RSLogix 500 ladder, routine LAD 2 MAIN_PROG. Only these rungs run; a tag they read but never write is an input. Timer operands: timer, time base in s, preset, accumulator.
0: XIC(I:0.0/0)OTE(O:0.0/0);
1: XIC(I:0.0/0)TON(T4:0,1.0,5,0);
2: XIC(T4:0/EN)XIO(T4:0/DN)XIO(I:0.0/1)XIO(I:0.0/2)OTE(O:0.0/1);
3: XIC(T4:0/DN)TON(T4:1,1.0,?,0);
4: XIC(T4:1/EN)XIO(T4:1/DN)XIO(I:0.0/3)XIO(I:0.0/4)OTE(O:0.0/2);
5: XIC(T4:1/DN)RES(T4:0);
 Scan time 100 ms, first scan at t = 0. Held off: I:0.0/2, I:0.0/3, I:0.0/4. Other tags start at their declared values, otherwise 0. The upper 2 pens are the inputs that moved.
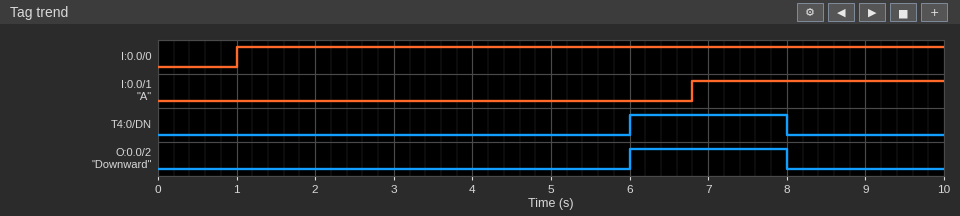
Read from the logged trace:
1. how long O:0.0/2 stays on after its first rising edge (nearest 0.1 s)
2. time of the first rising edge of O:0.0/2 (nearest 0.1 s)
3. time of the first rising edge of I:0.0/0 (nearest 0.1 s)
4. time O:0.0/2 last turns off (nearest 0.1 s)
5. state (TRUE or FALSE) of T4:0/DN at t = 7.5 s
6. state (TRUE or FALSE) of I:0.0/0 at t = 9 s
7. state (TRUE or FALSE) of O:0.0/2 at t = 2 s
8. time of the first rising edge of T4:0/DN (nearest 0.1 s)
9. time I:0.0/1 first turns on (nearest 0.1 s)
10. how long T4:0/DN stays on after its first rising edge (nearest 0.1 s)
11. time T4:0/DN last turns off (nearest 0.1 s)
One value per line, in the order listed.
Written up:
2.0 s
6.0 s
1.0 s
8.0 s
TRUE
TRUE
FALSE
6.0 s
6.8 s
2.0 s
8.0 s
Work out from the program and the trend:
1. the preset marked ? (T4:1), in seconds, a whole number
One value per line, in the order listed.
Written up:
2 s
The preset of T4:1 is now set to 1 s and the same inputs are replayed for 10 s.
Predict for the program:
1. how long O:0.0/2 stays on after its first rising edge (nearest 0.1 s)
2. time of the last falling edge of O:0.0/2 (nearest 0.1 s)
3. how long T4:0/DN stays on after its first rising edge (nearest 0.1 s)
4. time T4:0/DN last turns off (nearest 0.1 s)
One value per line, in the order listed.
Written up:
1.0 s
7.0 s
1.0 s
7.0 s
